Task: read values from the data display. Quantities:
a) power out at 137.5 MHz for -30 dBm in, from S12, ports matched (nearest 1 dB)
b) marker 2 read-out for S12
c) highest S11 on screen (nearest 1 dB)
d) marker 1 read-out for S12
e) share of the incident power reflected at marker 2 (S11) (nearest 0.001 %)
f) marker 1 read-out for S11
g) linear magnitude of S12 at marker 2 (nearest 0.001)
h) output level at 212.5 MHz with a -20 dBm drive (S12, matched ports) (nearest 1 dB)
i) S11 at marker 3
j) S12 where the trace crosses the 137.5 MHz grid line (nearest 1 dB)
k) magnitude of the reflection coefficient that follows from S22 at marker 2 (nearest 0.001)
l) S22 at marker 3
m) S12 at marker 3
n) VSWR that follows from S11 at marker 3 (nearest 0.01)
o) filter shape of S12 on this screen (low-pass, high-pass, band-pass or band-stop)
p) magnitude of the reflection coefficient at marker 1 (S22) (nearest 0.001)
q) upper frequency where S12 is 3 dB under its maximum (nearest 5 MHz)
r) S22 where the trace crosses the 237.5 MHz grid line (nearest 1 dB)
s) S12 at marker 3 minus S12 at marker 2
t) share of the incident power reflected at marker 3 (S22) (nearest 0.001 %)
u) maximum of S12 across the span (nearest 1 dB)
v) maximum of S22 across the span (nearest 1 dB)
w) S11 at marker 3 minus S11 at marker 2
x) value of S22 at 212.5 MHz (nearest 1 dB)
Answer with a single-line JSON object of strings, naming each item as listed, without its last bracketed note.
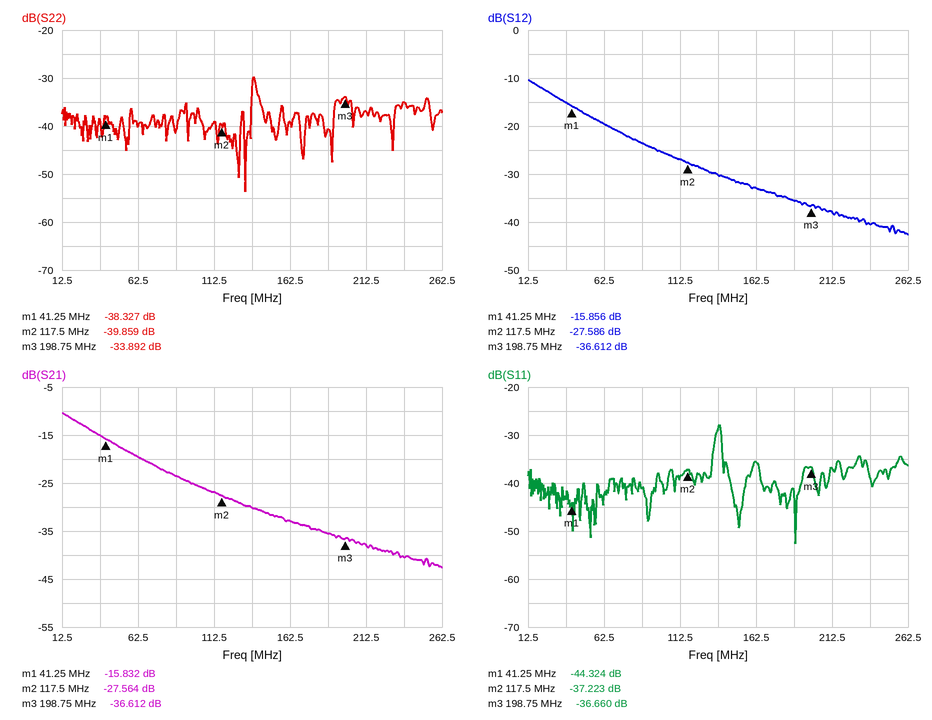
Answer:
{"power out at 137.5 MHz for -30 dBm in, from S12, ports matched": "-60 dBm", "marker 2 read-out for S12": "-27.586 dB", "highest S11 on screen": "-28 dB", "marker 1 read-out for S12": "-15.856 dB", "share of the incident power reflected at marker 2 (S11)": "0.019 %", "marker 1 read-out for S11": "-44.324 dB", "linear magnitude of S12 at marker 2": "0.042", "output level at 212.5 MHz with a -20 dBm drive (S12, matched ports)": "-58 dBm", "S11 at marker 3": "-36.660 dB", "S12 where the trace crosses the 137.5 MHz grid line": "-30 dB", "magnitude of the reflection coefficient that follows from S22 at marker 2": "0.010", "S22 at marker 3": "-33.892 dB", "S12 at marker 3": "-36.612 dB", "VSWR that follows from S11 at marker 3": "1.03", "filter shape of S12 on this screen": "low-pass", "magnitude of the reflection coefficient at marker 1 (S22)": "0.012", "upper frequency where S12 is 3 dB under its maximum": "30 MHz", "S22 where the trace crosses the 237.5 MHz grid line": "-35 dB", "S12 at marker 3 minus S12 at marker 2": "-9.026 dB", "share of the incident power reflected at marker 3 (S22)": "0.041 %", "maximum of S12 across the span": "-10 dB", "maximum of S22 across the span": "-30 dB", "S11 at marker 3 minus S11 at marker 2": "0.563 dB", "value of S22 at 212.5 MHz": "-37 dB"}
